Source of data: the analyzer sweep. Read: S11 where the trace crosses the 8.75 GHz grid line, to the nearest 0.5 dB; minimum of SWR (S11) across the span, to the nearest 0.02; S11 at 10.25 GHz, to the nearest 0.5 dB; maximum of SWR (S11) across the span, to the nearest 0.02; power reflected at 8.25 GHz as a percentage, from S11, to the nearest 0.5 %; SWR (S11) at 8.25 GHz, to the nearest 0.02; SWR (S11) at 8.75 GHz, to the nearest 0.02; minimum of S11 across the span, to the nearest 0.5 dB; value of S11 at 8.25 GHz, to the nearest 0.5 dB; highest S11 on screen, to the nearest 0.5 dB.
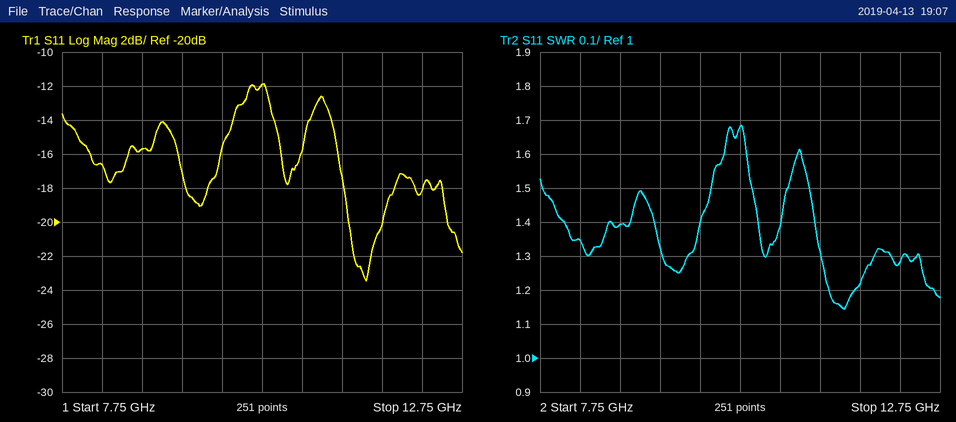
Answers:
-15.5 dB
1.14
-12.0 dB
1.68
2.0 %
1.34
1.40
-23.5 dB
-16.5 dB
-12.0 dB
